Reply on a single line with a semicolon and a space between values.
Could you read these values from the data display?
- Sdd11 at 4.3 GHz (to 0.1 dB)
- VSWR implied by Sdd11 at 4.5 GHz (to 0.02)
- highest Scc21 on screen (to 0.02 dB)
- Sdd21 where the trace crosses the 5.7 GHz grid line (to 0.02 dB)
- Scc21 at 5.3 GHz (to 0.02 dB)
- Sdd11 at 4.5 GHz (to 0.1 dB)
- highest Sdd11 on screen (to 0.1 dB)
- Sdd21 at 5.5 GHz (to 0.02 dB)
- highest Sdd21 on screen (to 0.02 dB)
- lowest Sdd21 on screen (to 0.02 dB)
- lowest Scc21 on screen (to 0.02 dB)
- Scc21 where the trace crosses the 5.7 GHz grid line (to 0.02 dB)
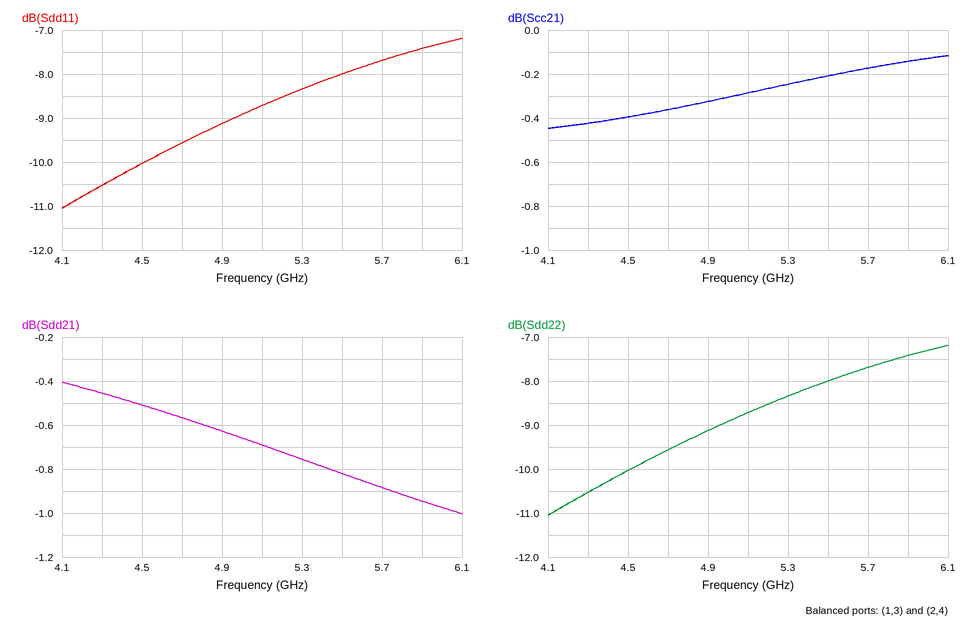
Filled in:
-10.5 dB; 1.92; -0.12 dB; -0.88 dB; -0.24 dB; -10.0 dB; -7.2 dB; -0.82 dB; -0.40 dB; -1.00 dB; -0.44 dB; -0.18 dB
